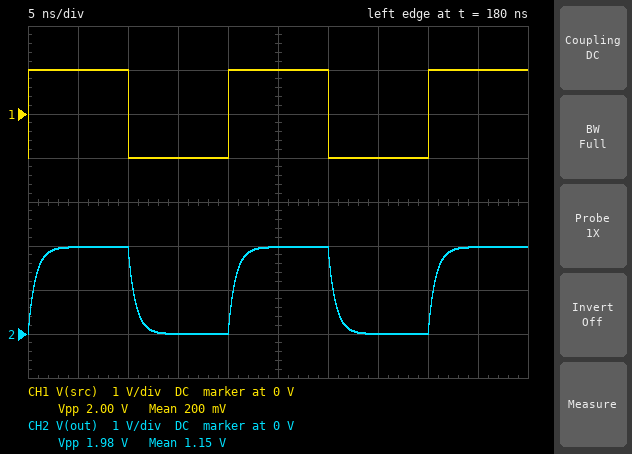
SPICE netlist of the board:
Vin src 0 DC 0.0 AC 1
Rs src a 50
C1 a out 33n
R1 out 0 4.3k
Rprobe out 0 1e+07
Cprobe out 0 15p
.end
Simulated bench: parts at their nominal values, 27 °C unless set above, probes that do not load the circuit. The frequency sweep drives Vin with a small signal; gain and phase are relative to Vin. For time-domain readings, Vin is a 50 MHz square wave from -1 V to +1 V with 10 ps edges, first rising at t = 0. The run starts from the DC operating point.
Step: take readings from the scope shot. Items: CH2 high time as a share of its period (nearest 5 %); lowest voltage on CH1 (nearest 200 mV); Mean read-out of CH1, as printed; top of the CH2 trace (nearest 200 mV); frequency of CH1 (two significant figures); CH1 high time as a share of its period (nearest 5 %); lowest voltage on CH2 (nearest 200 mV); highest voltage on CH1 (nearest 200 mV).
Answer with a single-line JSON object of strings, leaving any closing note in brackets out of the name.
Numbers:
{"CH2 high time as a share of its period": "50 %", "lowest voltage on CH1": "-1.0 V", "Mean read-out of CH1, as printed": "200 mV", "top of the CH2 trace": "2.0 V", "frequency of CH1": "50 MHz", "CH1 high time as a share of its period": "50 %", "lowest voltage on CH2": "0 V", "highest voltage on CH1": "1.0 V"}
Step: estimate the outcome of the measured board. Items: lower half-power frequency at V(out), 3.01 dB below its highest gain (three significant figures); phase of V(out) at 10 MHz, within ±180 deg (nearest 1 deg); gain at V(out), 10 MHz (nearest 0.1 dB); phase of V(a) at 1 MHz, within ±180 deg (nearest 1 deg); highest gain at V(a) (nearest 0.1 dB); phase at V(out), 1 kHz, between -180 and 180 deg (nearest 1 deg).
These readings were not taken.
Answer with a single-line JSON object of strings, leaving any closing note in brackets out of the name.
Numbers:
{"lower half-power frequency at V(out), 3.01 dB below its highest gain": "1.11 kHz", "phase of V(out) at 10 MHz, within ±180 deg": "-3 deg", "gain at V(out), 10 MHz": "-0.1 dB", "phase of V(a) at 1 MHz, within ±180 deg": "0 deg", "highest gain at V(a)": "0 dB", "phase at V(out), 1 kHz, between -180 and 180 deg": "48 deg"}
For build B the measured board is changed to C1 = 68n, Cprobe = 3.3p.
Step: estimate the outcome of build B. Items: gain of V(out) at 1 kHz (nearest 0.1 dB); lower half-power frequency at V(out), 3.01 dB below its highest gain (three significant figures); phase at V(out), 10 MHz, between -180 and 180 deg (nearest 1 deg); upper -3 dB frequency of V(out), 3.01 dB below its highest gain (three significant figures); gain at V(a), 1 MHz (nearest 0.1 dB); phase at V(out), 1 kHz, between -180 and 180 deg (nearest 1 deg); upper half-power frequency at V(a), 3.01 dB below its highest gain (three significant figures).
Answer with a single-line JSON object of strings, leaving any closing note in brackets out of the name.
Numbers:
{"gain of V(out) at 1 kHz": "-1.2 dB", "lower half-power frequency at V(out), 3.01 dB below its highest gain": "538 Hz", "phase at V(out), 10 MHz, between -180 and 180 deg": "-1 deg", "upper -3 dB frequency of V(out), 3.01 dB below its highest gain": "976 MHz", "gain at V(a), 1 MHz": "-0.1 dB", "phase at V(out), 1 kHz, between -180 and 180 deg": "28 deg", "upper half-power frequency at V(a), 3.01 dB below its highest gain": "953 MHz"}
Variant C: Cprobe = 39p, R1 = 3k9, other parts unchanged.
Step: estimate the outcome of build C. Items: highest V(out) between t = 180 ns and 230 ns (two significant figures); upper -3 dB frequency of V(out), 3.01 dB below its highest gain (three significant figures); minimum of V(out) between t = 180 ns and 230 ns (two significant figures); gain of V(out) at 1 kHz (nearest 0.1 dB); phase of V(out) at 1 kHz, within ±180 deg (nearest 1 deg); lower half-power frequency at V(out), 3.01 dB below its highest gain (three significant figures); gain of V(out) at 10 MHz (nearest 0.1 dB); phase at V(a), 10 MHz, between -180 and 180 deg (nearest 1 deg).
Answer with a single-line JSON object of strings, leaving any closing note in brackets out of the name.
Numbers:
{"highest V(out) between t = 180 ns and 230 ns": "2.0 V", "upper -3 dB frequency of V(out), 3.01 dB below its highest gain": "82.8 MHz", "minimum of V(out) between t = 180 ns and 230 ns": "9.2 mV", "gain of V(out) at 1 kHz": "-4.1 dB", "phase of V(out) at 1 kHz, within ±180 deg": "51 deg", "lower half-power frequency at V(out), 3.01 dB below its highest gain": "1.22 kHz", "gain of V(out) at 10 MHz": "-0.2 dB", "phase at V(a), 10 MHz, between -180 and 180 deg": "-7 deg"}
